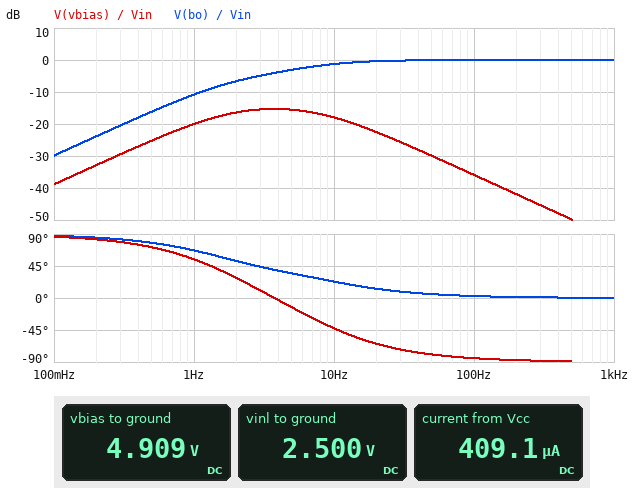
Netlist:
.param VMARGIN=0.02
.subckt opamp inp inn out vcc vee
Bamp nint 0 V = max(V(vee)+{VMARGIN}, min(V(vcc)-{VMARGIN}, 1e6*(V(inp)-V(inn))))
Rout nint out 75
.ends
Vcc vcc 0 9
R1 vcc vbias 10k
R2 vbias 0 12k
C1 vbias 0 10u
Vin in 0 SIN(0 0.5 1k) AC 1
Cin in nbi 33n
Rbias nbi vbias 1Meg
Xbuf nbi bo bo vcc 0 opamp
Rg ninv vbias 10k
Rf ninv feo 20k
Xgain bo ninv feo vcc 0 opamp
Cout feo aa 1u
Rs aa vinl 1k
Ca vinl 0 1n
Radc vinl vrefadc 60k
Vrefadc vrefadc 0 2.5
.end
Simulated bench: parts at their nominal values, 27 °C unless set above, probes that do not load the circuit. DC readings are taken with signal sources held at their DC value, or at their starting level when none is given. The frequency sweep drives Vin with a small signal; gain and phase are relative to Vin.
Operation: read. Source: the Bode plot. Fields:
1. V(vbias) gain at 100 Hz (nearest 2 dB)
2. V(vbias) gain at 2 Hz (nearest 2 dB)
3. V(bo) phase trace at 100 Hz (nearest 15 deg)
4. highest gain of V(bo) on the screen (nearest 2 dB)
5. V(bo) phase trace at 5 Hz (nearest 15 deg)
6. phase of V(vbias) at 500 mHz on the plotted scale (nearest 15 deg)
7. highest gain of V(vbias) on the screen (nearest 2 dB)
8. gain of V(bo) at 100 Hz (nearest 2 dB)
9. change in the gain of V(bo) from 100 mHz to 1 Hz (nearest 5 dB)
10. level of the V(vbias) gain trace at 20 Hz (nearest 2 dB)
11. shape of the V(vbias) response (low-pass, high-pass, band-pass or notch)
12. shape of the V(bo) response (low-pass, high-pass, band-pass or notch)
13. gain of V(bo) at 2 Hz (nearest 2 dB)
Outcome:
-36 dB
-16 dB
0 deg
0 dB
30 deg
75 deg
-16 dB
0 dB
20 dB
-22 dB
band-pass
high-pass
-6 dB
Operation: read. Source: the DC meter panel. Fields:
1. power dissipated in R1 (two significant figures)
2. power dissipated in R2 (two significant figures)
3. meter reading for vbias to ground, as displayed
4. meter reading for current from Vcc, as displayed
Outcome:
1.7 mW
2.0 mW
4.909 V
409.1 µA
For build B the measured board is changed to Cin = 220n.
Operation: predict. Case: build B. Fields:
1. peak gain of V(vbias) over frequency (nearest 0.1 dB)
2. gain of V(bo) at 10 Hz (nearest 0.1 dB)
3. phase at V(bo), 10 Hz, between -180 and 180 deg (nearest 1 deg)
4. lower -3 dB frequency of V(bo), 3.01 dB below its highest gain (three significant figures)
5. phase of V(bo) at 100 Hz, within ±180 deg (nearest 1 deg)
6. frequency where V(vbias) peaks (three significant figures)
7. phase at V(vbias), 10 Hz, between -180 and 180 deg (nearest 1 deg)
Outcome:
-10.3 dB
-0.1 dB
4 deg
499 mHz
0 deg
1.45 Hz
-62 deg
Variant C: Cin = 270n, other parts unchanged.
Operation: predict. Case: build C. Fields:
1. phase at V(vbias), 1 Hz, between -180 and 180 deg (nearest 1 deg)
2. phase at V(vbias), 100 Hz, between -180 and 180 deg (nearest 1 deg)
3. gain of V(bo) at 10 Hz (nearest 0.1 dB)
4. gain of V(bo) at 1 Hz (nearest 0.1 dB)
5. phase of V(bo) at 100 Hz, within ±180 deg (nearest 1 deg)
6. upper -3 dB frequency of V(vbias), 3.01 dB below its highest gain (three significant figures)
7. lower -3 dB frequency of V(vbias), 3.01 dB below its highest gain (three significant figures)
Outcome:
8 deg
-87 deg
-0.1 dB
-0.9 dB
0 deg
5.43 Hz
317 mHz
